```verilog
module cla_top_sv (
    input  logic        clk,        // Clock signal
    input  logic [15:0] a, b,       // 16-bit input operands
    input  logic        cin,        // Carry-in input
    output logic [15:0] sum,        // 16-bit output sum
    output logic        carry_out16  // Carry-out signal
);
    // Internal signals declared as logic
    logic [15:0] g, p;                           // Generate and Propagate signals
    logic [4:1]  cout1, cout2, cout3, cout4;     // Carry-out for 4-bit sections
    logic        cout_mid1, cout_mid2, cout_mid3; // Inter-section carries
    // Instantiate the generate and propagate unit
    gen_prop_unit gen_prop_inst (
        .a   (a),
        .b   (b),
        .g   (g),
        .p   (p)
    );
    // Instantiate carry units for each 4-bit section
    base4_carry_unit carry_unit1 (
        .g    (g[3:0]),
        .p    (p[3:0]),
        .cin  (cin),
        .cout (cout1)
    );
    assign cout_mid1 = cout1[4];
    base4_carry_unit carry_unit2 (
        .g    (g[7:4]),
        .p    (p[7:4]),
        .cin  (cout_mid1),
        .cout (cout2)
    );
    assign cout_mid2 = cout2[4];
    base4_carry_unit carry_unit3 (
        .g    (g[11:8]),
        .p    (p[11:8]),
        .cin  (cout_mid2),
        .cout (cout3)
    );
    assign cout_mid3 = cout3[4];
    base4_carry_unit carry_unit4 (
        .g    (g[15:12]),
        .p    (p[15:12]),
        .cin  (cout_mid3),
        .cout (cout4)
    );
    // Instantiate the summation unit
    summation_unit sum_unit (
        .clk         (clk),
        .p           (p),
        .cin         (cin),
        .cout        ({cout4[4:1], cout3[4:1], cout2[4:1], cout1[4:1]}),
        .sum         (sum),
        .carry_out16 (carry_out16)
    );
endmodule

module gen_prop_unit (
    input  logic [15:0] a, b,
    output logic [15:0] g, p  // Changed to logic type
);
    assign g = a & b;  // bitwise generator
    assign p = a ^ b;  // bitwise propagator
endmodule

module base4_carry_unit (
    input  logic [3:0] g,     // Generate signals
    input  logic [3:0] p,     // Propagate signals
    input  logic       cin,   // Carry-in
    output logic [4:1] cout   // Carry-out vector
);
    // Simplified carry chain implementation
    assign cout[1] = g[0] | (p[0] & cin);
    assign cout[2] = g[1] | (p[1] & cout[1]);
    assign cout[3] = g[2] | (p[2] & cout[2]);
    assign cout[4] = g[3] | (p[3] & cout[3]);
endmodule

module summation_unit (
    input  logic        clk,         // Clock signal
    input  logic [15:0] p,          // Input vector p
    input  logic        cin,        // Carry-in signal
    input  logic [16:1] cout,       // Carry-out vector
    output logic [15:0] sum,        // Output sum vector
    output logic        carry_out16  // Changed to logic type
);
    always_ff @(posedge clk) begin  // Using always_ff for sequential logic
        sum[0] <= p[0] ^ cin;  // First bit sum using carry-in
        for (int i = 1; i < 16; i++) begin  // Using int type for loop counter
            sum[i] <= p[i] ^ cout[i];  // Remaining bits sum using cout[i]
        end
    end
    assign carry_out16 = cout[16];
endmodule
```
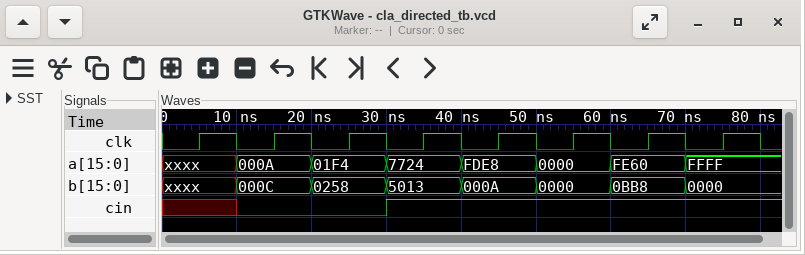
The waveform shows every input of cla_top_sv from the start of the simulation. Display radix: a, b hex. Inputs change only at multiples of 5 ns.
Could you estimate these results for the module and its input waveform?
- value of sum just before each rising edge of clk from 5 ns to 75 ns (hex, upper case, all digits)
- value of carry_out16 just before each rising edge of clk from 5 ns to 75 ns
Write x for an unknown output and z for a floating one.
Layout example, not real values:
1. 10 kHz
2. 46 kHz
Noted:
1. x, x, 0016, 044C, C738, FDF3, 0001, 0A19
2. x 0 0 0 0 0 1 1
